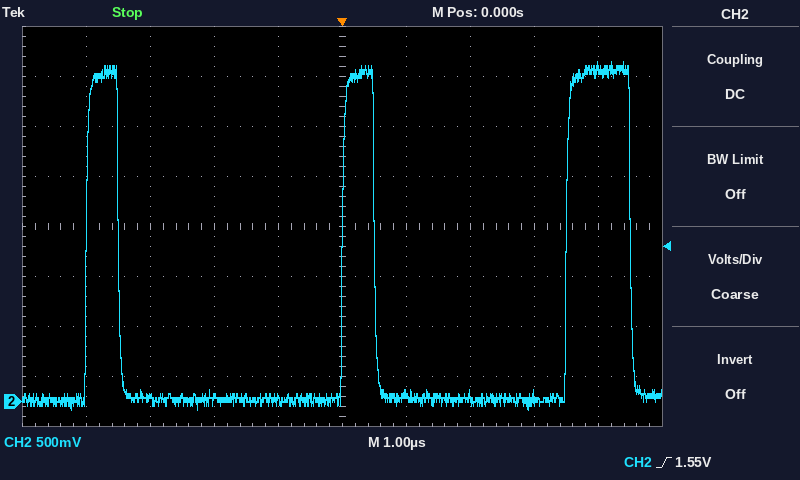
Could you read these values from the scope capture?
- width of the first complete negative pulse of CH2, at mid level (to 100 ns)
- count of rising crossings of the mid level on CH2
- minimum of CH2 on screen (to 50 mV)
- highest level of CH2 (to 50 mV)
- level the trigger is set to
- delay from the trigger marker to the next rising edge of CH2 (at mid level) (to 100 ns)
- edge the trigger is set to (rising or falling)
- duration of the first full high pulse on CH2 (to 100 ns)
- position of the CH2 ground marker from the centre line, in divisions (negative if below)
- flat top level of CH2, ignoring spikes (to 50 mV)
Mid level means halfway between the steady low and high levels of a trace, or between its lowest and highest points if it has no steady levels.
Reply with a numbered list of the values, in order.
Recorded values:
1. 3.5 µs
2. 3
3. -100 mV
4. 3.40 V
5. 1.55 V
6. 3.5 µs
7. rising
8. 500 ns
9. -3.5 div
10. 3.30 V
